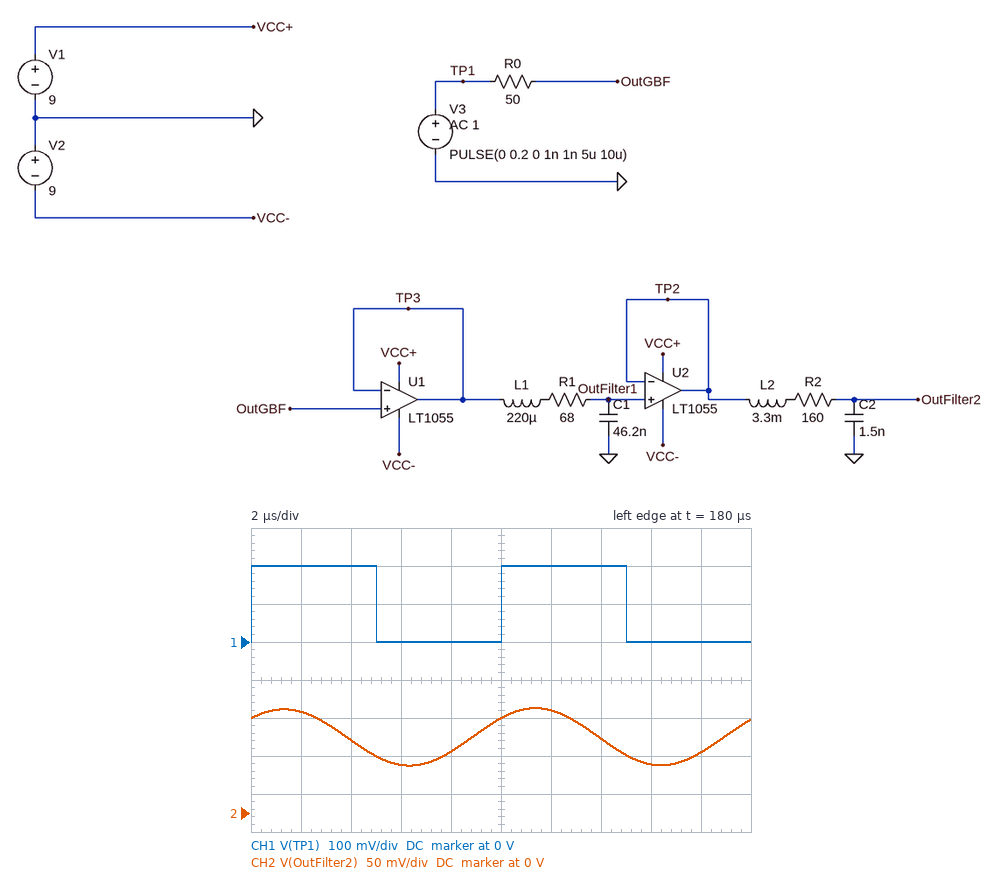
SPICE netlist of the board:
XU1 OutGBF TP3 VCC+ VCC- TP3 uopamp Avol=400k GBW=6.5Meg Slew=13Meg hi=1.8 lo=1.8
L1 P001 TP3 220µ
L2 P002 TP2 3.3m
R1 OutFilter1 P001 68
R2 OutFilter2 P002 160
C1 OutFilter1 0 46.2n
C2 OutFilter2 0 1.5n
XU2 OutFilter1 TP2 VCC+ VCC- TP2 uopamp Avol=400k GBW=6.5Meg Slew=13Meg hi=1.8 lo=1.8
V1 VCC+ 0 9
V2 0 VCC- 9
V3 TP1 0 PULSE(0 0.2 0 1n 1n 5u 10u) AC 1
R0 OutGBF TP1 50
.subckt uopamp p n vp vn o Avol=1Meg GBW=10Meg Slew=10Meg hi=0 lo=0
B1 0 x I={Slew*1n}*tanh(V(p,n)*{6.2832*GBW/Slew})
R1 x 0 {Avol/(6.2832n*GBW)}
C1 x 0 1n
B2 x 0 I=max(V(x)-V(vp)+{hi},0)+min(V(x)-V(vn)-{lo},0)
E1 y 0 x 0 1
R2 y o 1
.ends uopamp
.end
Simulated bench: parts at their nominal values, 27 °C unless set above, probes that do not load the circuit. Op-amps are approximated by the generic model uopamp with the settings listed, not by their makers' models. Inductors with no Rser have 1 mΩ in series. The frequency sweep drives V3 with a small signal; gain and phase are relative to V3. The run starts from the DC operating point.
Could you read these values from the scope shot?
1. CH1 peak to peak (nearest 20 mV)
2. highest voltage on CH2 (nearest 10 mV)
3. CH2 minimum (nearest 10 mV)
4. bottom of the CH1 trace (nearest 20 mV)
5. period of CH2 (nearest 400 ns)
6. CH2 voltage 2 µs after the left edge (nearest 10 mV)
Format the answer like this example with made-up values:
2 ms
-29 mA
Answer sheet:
200 mV
140 mV
60 mV
0 V
10.0 µs
130 mV
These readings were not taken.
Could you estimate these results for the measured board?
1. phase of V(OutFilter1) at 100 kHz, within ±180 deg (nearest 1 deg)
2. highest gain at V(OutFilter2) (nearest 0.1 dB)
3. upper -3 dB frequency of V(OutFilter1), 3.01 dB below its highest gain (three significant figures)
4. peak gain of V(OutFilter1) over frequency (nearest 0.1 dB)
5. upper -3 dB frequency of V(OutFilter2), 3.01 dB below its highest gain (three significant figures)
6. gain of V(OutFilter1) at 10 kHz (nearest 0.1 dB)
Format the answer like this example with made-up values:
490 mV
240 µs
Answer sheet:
-148 deg
14.5 dB
58.5 kHz
1.3 dB
74.4 kHz
0.2 dB
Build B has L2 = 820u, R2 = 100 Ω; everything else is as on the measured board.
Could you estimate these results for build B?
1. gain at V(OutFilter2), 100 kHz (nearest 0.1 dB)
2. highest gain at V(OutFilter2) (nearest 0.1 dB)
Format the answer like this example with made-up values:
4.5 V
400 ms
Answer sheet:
-5.5 dB
1.9 dB
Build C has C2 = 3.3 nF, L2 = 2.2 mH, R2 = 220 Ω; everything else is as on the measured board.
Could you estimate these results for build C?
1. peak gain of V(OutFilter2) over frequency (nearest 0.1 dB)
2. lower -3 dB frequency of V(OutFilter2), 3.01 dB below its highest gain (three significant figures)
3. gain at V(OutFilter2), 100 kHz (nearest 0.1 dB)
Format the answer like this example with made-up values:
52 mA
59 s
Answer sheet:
10.1 dB
43.8 kHz
-16.8 dB
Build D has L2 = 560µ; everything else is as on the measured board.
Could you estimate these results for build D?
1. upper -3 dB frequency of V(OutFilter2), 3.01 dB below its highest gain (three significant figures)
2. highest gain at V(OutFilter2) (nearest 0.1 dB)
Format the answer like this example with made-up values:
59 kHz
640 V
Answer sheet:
61.5 kHz
1.7 dB
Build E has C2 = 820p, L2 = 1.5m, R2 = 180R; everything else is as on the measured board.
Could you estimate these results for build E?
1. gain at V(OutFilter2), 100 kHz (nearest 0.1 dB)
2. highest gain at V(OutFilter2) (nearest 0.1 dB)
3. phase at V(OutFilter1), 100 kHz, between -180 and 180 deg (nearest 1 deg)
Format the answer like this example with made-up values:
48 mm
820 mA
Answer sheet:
-5.5 dB
1.9 dB
-148 deg
